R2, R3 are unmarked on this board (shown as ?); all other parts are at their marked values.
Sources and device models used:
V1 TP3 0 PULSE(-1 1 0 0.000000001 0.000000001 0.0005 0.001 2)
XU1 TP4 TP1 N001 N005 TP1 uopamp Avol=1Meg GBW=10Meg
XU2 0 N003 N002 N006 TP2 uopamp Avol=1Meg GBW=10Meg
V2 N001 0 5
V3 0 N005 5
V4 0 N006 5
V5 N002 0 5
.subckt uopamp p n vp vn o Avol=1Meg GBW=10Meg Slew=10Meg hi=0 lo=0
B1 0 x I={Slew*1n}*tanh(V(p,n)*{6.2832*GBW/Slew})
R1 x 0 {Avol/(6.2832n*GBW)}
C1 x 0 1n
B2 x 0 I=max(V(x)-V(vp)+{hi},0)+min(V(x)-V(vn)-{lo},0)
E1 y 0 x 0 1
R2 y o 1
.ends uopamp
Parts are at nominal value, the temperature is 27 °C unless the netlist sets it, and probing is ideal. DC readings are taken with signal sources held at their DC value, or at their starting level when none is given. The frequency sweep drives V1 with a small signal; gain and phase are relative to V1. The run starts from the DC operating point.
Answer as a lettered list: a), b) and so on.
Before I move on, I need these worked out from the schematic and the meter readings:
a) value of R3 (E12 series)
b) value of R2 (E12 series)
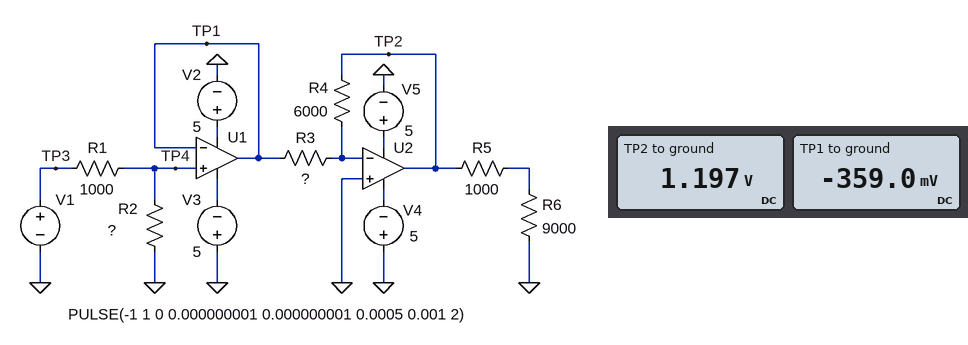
a) 1.8 kΩ
b) 560 Ω
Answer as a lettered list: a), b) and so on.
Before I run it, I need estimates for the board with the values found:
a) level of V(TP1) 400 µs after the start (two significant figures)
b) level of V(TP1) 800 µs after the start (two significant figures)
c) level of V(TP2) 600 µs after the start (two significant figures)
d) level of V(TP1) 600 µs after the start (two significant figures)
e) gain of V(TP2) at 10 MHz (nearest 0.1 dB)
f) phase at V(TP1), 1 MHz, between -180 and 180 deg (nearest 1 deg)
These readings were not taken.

a) 360 mV
b) -360 mV
c) 1.2 V
d) -360 mV
e) -14.4 dB
f) -6 deg
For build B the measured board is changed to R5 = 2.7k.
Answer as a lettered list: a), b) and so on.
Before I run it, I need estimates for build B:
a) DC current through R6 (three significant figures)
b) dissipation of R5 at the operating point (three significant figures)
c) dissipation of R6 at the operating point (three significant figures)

a) 102 µA
b) 28.2 µW
c) 94.1 µW
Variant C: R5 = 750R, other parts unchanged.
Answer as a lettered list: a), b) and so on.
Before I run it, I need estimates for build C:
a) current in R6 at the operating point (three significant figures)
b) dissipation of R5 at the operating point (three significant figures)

a) 123 µA
b) 11.3 µW
